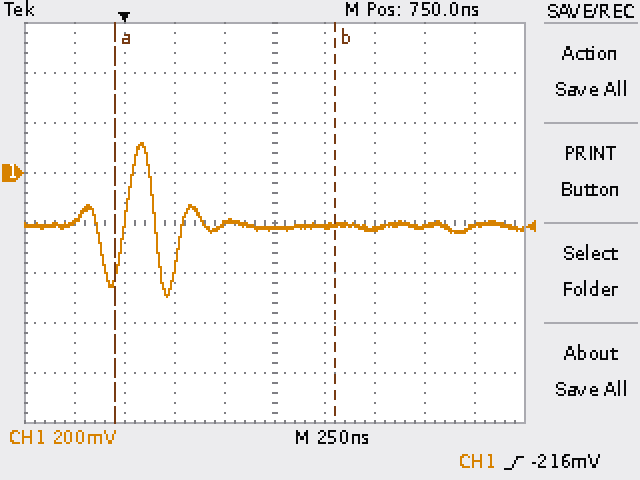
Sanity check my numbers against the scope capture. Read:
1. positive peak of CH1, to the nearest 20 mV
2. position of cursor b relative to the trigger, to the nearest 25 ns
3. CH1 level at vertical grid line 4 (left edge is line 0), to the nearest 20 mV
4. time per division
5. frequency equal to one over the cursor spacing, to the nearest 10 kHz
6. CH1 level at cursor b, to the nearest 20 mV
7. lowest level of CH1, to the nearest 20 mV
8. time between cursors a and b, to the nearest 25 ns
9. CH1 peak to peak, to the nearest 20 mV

120 mV
+1.050 µs
-200 mV
250 ns
910 kHz
-220 mV
-500 mV
1.100 µs
620 mV
